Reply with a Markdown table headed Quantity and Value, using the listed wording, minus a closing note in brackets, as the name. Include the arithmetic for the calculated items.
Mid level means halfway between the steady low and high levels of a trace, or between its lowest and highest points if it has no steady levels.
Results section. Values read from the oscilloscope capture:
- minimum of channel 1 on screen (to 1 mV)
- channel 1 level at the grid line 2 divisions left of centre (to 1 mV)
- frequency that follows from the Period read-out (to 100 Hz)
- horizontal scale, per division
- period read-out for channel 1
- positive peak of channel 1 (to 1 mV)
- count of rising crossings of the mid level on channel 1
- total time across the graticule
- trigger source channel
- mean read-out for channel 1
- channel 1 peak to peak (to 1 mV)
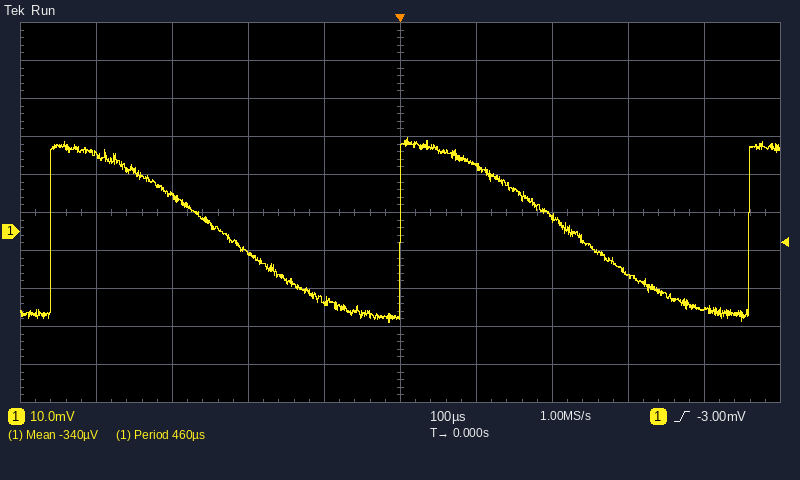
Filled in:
| Quantity | Value |
|---|---|
| minimum of channel 1 on screen | -24 mV |
| channel 1 level at the grid line 2 divisions left of centre | -6 mV |
| frequency that follows from the Period read-out | 1 / 460 µs ≈ 2.2 kHz |
| horizontal scale, per division | 100 µs |
| period read-out for channel 1 | 460 µs |
| positive peak of channel 1 | 25 mV |
| count of rising crossings of the mid level on channel 1 | 3 |
| total time across the graticule | 1 ms |
| trigger source channel | channel 1 |
| mean read-out for channel 1 | -340 µV |
| channel 1 peak to peak | 25 mV − (-24 mV) = 49 mV |
